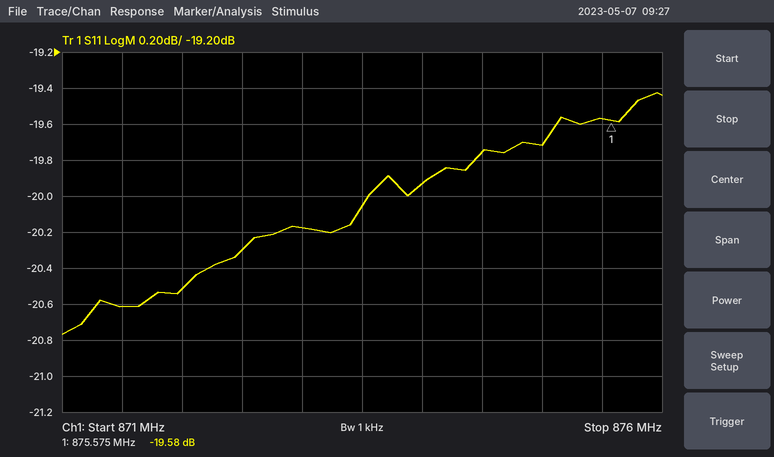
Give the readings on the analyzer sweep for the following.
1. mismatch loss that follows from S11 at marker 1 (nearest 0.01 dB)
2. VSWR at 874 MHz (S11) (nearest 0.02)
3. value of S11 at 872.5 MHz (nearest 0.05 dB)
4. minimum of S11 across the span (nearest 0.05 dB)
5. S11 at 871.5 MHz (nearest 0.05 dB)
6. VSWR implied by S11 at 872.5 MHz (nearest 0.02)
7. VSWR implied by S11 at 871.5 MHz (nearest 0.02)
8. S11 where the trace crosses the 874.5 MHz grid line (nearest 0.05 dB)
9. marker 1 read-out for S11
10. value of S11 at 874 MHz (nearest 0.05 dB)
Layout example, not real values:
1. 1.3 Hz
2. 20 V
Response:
1. 0.05 dB
2. 1.22
3. -20.30 dB
4. -20.75 dB
5. -20.60 dB
6. 1.22
7. 1.20
8. -19.75 dB
9. -19.58 dB
10. -19.95 dB
